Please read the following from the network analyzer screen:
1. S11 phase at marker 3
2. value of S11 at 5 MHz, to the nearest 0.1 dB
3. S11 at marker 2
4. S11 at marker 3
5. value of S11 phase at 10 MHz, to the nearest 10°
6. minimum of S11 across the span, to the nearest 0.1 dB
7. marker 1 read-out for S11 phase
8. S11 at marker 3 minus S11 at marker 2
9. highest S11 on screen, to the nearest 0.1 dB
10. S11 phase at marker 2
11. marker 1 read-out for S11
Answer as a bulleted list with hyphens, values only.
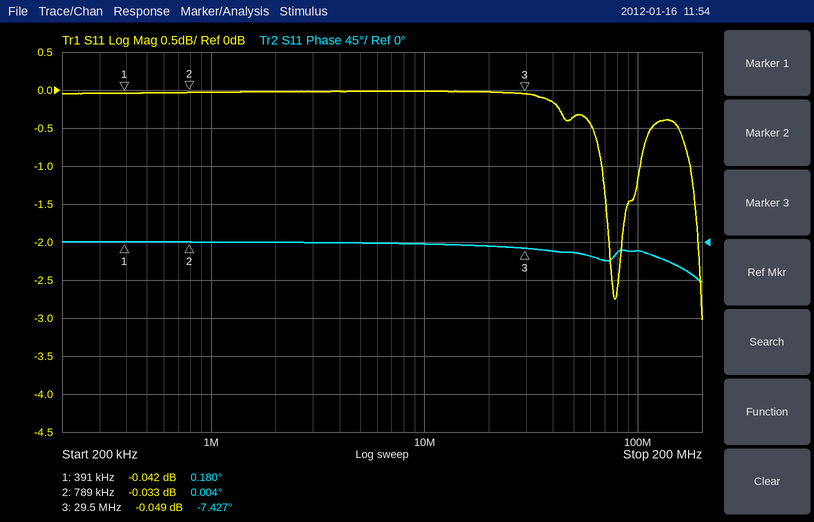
- -7.427°
- 0.0 dB
- -0.033 dB
- -0.049 dB
- 0°
- -3.0 dB
- 0.180°
- -0.016 dB
- 0.0 dB
- 0.004°
- -0.042 dB
